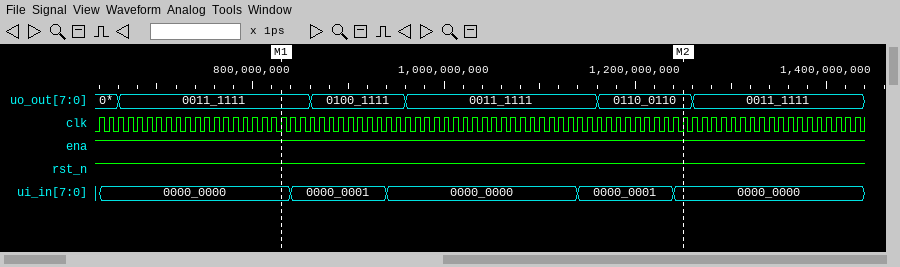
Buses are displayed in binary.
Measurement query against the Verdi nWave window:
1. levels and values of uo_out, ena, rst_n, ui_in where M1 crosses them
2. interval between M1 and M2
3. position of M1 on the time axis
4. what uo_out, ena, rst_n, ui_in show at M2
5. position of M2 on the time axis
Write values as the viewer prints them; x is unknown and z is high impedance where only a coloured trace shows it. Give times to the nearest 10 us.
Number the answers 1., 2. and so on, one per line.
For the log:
1. uo_out=0011_1111, ena=1, rst_n=1, ui_in=0000_0000
2. 420 us
3. 830 us
4. uo_out=0110_0110, ena=1, rst_n=1, ui_in=0000_0000
5. 1250 us
